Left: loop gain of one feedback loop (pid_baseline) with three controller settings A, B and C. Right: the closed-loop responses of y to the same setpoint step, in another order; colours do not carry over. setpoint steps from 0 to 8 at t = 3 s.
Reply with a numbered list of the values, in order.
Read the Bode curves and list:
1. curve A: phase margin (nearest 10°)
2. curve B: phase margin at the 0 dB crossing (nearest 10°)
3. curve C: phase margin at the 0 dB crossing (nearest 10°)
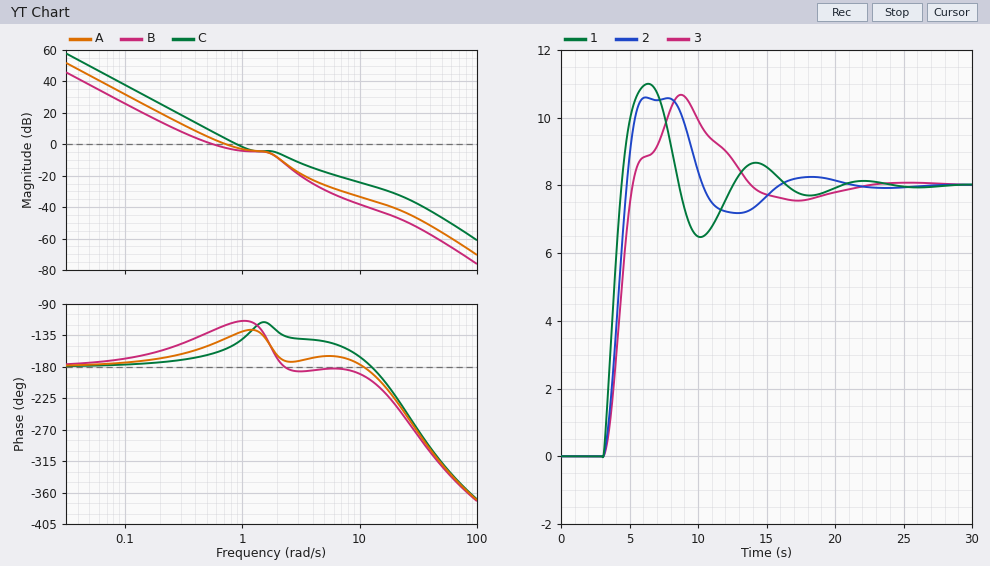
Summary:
1. 40°
2. 50°
3. 30°
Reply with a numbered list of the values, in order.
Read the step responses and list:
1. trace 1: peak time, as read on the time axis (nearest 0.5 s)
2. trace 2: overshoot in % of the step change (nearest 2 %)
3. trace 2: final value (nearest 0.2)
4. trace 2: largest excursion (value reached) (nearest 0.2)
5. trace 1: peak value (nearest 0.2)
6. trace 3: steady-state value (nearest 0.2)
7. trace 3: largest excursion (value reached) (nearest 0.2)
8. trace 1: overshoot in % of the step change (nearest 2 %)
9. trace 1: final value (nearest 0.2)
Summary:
1. 6.5 s
2. 32 %
3. 8.0
4. 10.6
5. 11.0
6. 8.0
7. 10.6
8. 38 %
9. 8.0
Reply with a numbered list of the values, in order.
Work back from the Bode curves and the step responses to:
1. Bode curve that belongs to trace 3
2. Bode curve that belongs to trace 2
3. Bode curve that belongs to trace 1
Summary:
1. B
2. A
3. C
